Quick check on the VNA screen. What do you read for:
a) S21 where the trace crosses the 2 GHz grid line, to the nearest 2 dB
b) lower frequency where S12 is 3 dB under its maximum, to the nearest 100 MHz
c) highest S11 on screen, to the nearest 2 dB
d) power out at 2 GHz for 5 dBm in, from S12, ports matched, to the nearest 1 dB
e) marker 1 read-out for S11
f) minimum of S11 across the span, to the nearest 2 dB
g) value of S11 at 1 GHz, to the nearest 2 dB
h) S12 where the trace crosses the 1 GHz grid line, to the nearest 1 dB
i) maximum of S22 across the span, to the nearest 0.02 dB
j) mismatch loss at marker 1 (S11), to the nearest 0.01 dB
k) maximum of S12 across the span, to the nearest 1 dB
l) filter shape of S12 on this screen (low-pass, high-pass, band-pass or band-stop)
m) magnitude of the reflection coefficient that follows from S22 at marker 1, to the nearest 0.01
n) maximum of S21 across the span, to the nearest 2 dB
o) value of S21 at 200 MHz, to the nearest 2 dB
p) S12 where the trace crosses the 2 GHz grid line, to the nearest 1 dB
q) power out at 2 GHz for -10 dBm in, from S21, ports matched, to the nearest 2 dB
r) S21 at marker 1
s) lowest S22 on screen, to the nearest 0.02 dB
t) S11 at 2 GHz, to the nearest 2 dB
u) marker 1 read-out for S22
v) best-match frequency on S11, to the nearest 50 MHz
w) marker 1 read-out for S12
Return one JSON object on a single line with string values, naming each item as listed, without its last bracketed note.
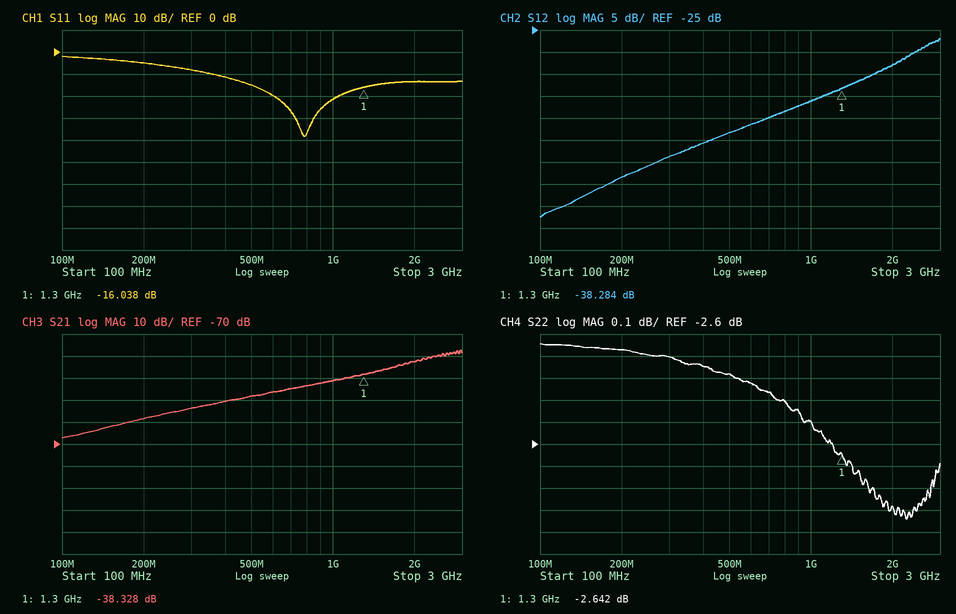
{"S21 where the trace crosses the 2 GHz grid line, to the nearest 2 dB": "-32 dB", "lower frequency where S12 is 3 dB under its maximum, to the nearest 100 MHz": "2.4 GHz", "highest S11 on screen, to the nearest 2 dB": "-2 dB", "power out at 2 GHz for 5 dBm in, from S12, ports matched, to the nearest 1 dB": "-28 dBm", "marker 1 read-out for S11": "-16.038 dB", "minimum of S11 across the span, to the nearest 2 dB": "-38 dB", "value of S11 at 1 GHz, to the nearest 2 dB": "-22 dB", "S12 where the trace crosses the 1 GHz grid line, to the nearest 1 dB": "-41 dB", "maximum of S22 across the span, to the nearest 0.02 dB": "-2.14 dB", "mismatch loss at marker 1 (S11), to the nearest 0.01 dB": "0.11 dB", "maximum of S12 across the span, to the nearest 1 dB": "-27 dB", "filter shape of S12 on this screen": "high-pass", "magnitude of the reflection coefficient that follows from S22 at marker 1, to the nearest 0.01": "0.74", "maximum of S21 across the span, to the nearest 2 dB": "-28 dB", "value of S21 at 200 MHz, to the nearest 2 dB": "-58 dB", "S12 where the trace crosses the 2 GHz grid line, to the nearest 1 dB": "-33 dB", "power out at 2 GHz for -10 dBm in, from S21, ports matched, to the nearest 2 dB": "-42 dBm", "S21 at marker 1": "-38.328 dB", "lowest S22 on screen, to the nearest 0.02 dB": "-2.94 dB", "S11 at 2 GHz, to the nearest 2 dB": "-14 dB", "marker 1 read-out for S22": "-2.642 dB", "best-match frequency on S11, to the nearest 50 MHz": "800 MHz", "marker 1 read-out for S12": "-38.284 dB"}
